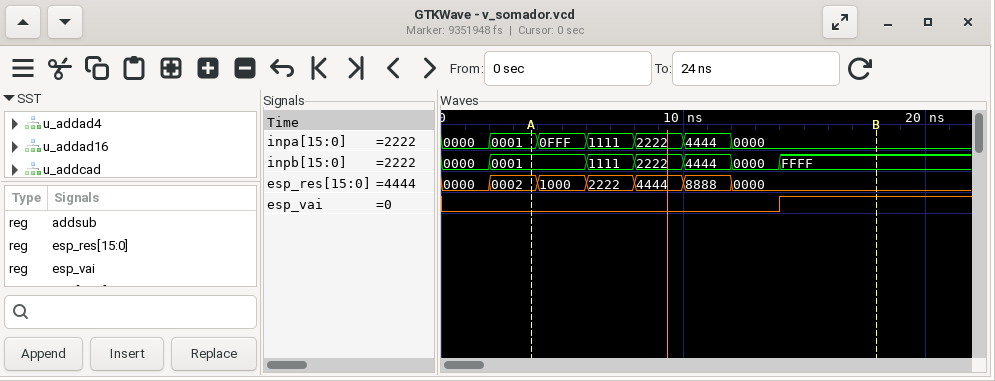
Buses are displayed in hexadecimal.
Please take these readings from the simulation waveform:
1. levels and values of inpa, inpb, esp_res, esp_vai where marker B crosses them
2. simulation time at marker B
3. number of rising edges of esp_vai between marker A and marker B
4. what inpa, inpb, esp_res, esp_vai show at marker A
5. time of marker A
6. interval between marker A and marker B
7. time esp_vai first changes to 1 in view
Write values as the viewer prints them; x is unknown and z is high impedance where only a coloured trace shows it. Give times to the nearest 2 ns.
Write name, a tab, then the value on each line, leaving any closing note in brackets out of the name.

levels and values of inpa, inpb, esp_res, esp_vai where marker B crosses them	inpa=0000, inpb=FFFF, esp_res=0000, esp_vai=1
simulation time at marker B	18 ns
number of rising edges of esp_vai between marker A and marker B	1
what inpa, inpb, esp_res, esp_vai show at marker A	inpa=0001, inpb=0001, esp_res=0002, esp_vai=0
time of marker A	4 ns
interval between marker A and marker B	14 ns
time esp_vai first changes to 1 in view	14 ns
